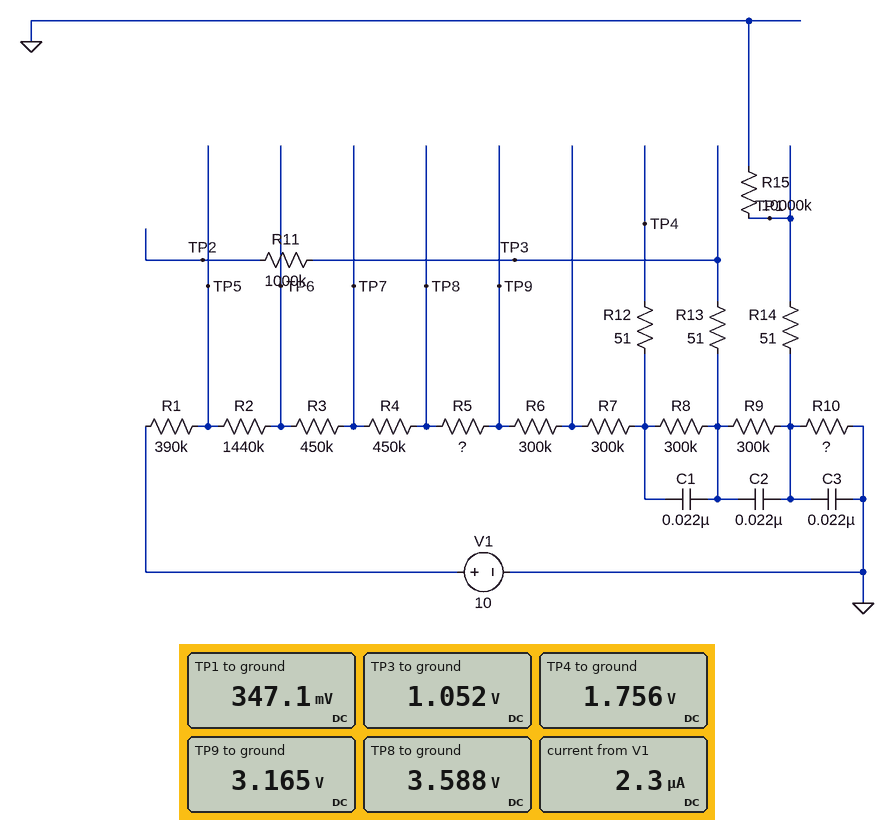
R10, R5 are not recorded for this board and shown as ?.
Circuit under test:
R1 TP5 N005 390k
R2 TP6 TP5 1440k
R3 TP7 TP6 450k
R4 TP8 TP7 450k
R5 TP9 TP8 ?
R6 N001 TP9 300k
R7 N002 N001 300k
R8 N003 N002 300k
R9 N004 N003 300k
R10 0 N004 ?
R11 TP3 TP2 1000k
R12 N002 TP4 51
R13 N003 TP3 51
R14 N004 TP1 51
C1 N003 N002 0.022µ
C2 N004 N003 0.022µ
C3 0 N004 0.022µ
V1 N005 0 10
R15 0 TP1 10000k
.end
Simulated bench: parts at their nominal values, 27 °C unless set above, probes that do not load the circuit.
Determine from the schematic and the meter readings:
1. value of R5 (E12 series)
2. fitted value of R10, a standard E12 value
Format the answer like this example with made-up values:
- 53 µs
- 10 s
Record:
- 180 kΩ
- 150 kΩ
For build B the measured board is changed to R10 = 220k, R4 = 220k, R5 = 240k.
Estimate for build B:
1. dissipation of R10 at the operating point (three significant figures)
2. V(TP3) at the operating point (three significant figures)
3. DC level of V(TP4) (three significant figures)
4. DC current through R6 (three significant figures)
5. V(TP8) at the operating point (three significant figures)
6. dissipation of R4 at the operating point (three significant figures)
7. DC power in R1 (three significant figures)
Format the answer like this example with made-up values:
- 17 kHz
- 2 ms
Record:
- 1.22 µW
- 1.24 V
- 1.96 V
- 2.41 µA
- 3.98 V
- 1.27 µW
- 2.26 µW
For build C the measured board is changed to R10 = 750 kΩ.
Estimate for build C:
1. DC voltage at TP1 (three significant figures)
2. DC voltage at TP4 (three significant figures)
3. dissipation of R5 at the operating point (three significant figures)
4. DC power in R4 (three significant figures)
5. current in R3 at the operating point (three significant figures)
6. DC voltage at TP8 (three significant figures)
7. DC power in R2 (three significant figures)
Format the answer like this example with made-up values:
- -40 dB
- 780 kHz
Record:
- 1.45 V
- 2.70 V
- 779 nW
- 1.95 µW
- 2.08 µA
- 4.32 V
- 6.23 µW
